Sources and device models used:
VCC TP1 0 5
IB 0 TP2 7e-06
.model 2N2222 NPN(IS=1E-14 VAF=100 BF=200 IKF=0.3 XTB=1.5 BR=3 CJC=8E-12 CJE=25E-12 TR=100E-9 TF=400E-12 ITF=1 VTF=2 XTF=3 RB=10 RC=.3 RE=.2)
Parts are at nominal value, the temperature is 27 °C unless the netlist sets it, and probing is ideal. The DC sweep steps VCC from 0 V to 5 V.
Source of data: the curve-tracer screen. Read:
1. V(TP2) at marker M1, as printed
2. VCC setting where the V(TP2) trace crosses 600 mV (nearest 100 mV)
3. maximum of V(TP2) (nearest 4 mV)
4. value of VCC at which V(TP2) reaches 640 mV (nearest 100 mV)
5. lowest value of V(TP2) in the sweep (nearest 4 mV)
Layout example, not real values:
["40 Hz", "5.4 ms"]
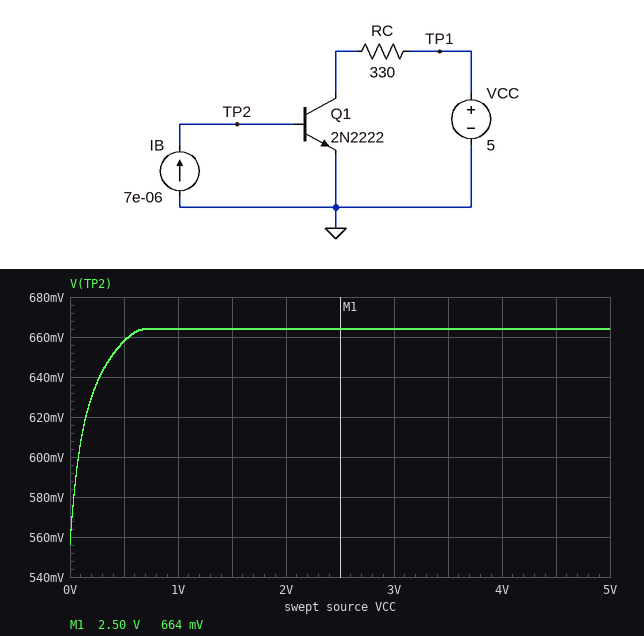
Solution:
["664 mV", "100 mV", "664 mV", "300 mV", "556 mV"]
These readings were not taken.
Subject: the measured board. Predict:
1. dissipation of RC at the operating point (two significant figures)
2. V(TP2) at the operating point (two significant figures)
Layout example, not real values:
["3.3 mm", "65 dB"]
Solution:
["690 µW", "660 mV"]
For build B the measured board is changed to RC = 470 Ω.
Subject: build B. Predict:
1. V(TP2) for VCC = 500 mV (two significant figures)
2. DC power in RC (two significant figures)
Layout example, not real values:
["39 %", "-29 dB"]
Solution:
["650 mV", "980 µW"]
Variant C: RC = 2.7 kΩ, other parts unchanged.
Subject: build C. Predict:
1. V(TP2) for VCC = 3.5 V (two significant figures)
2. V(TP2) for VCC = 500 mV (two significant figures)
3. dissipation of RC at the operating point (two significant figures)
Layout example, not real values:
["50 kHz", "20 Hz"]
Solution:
["660 mV", "610 mV", "5.3 mW"]
